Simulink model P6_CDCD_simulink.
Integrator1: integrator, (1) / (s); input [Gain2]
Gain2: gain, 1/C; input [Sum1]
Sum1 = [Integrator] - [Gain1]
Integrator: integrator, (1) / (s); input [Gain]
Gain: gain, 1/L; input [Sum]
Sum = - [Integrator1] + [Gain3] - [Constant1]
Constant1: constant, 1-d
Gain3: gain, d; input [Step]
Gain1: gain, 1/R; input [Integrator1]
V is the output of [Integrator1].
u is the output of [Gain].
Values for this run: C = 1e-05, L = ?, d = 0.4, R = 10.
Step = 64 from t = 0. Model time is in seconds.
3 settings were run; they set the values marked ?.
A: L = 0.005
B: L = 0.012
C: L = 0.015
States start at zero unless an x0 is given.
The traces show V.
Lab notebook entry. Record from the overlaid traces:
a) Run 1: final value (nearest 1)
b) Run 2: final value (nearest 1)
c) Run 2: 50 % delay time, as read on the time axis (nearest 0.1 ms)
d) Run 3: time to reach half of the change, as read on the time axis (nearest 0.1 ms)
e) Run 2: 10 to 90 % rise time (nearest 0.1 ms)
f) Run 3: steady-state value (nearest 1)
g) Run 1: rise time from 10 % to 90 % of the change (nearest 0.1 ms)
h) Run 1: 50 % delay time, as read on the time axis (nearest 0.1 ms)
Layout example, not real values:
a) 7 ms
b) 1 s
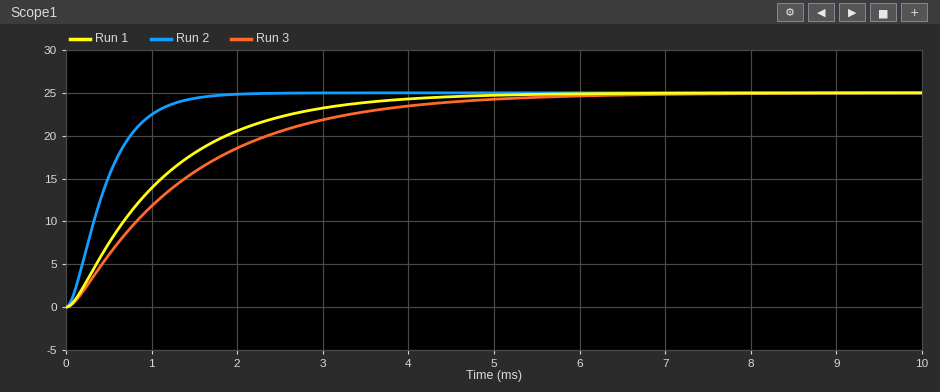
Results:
a) 25
b) 25
c) 0.4 ms
d) 1.1 ms
e) 0.9 ms
f) 25
g) 2.4 ms
h) 0.9 ms
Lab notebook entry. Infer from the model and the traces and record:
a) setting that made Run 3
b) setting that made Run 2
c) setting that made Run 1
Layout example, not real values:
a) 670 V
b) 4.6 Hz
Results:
a) C
b) A
c) B
